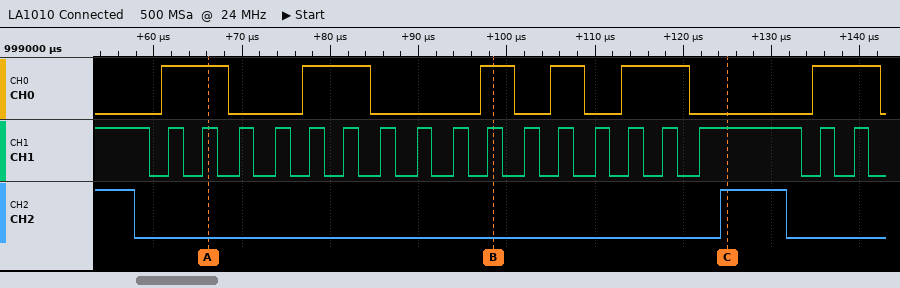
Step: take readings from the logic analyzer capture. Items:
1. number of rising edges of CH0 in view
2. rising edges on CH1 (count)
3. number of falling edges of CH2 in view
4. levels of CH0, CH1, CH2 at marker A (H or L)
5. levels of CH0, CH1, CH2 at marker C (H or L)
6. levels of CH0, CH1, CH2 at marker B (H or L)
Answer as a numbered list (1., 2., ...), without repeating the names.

1. 6
2. 18
3. 2
4. CH0=H, CH1=H, CH2=L
5. CH0=L, CH1=H, CH2=H
6. CH0=H, CH1=H, CH2=L
